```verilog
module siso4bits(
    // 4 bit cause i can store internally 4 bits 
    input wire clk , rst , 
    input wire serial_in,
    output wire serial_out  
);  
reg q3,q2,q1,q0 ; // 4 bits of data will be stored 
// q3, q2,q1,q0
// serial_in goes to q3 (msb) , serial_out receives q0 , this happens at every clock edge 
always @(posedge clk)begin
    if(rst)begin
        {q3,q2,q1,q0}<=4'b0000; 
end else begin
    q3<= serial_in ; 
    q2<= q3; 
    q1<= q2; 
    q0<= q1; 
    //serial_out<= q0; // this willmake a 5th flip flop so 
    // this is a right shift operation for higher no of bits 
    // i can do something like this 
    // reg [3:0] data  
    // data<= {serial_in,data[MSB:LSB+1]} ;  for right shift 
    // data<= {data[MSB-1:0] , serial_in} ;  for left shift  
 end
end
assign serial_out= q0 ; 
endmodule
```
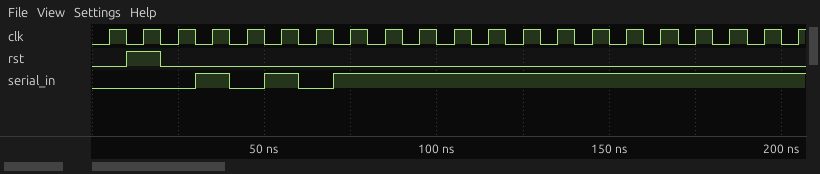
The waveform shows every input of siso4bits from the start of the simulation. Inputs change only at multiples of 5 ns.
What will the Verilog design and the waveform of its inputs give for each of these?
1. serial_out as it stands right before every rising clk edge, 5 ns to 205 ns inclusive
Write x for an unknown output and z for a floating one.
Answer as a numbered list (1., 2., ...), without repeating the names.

1. x x 0 0 0 0 0 1 0 1 0 1 1 1 1 1 1 1 1 1 1
